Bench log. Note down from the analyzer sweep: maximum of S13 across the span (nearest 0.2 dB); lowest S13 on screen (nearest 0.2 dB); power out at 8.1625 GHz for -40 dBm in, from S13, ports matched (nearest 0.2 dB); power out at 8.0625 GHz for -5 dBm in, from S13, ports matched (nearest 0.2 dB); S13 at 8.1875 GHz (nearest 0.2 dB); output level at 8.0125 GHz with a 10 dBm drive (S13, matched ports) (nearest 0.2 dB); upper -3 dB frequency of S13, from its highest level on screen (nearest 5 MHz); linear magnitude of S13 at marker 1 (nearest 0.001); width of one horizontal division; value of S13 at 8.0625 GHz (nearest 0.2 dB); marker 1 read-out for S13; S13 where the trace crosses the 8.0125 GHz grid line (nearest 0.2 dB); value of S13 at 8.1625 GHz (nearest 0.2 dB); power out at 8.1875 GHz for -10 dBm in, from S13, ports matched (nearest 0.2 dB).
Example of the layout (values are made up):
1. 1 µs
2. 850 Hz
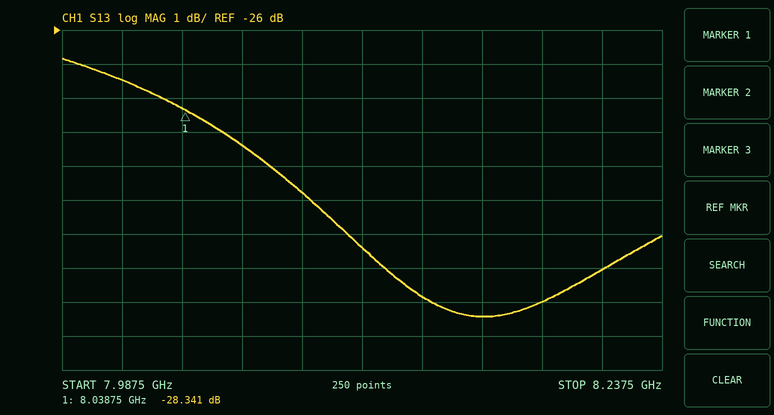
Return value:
1. -26.8 dB
2. -34.4 dB
3. -74.4 dBm
4. -34.4 dBm
5. -34.0 dB
6. -17.4 dBm
7. 8.070 GHz
8. 0.038
9. 25 MHz
10. -29.4 dB
11. -28.341 dB
12. -27.4 dB
13. -34.4 dB
14. -44.0 dBm
